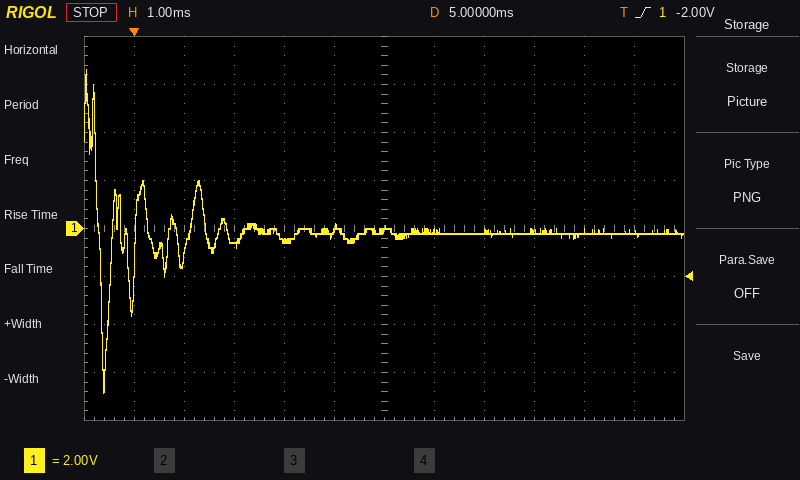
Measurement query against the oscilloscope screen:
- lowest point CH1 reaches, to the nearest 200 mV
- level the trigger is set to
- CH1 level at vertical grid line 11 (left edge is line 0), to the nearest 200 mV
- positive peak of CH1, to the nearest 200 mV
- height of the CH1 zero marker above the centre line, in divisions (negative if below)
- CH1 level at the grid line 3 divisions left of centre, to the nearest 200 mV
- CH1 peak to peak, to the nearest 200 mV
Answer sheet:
-6.8 V
-2.00 V
-200 mV
6.6 V
0.0 div
-600 mV
13.4 V
